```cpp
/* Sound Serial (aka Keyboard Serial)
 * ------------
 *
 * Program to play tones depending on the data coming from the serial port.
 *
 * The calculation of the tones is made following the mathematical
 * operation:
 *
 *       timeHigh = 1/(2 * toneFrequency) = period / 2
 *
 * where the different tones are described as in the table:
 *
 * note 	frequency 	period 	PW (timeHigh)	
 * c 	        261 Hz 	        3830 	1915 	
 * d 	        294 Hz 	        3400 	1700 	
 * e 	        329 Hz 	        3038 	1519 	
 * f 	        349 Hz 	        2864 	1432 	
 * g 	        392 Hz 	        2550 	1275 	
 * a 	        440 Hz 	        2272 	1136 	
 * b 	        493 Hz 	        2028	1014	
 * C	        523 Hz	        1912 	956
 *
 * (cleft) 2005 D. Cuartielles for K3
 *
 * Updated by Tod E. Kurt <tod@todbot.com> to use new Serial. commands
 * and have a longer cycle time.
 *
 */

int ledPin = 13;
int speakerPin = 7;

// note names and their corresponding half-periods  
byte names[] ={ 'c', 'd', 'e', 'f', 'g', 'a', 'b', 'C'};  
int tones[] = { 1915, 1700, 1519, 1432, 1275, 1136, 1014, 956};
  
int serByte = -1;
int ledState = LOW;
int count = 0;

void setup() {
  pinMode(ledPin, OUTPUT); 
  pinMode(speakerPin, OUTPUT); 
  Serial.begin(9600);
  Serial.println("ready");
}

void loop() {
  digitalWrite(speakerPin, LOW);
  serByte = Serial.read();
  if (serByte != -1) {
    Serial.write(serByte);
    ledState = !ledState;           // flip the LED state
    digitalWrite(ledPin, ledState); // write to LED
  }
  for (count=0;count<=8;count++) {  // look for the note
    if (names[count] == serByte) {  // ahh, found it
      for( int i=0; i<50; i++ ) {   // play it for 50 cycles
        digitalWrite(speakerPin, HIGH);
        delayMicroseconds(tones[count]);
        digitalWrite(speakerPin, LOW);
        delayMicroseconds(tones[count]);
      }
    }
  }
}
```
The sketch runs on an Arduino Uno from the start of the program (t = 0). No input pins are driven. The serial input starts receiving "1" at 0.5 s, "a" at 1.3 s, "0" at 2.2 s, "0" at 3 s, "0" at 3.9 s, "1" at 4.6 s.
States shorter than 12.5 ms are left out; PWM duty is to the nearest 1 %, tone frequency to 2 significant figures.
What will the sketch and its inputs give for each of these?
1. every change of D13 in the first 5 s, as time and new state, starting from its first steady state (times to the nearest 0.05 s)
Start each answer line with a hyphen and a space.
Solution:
- 0 s low; 0.5 s high; 1.3 s low; 2.2 s high; 3 s low; 3.9 s high; 4.6 s low
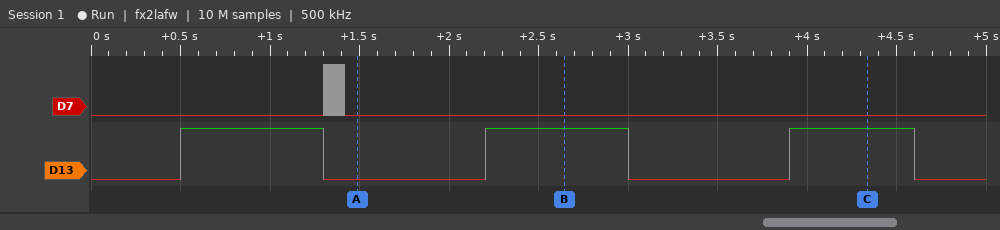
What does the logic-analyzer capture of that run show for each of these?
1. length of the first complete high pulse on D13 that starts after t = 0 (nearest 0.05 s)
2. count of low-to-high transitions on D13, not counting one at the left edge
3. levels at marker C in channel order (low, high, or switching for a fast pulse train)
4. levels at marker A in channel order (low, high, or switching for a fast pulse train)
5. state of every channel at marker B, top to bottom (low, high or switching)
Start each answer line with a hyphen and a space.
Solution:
- 0.80 s
- 3
- D7 low, D13 high
- D7 low, D13 low
- D7 low, D13 high
